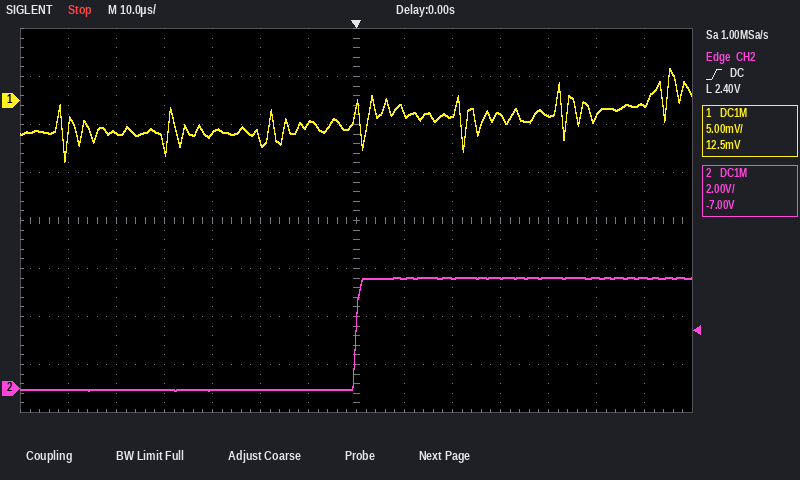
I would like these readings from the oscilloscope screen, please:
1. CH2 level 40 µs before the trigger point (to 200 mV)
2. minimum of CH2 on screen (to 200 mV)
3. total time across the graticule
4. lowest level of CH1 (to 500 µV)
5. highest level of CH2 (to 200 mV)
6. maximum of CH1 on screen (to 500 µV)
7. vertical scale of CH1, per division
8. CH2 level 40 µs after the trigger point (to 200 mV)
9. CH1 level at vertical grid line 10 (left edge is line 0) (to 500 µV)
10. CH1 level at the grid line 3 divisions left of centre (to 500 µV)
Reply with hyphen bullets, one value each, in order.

- 0.0 V
- 0.0 V
- 140 µs
- -6.5 mV
- 4.6 V
- 3.5 mV
- 5 mV
- 4.6 V
- -1.5 mV
- -3.5 mV
